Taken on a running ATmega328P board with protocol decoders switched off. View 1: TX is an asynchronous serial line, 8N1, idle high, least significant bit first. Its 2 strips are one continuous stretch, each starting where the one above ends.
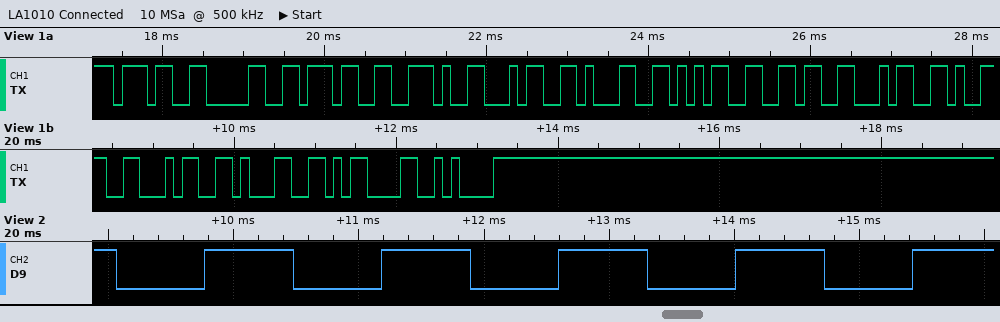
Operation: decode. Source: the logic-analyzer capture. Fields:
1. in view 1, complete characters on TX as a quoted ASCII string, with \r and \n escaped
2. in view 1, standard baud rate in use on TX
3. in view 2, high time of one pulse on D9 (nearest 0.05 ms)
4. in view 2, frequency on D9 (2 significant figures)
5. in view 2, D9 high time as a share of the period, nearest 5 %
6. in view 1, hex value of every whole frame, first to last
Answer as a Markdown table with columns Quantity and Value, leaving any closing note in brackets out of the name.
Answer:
| Quantity | Value |
|---|---|
| in view 1, complete characters on TX as a quoted ASCII string, with \r and \n escaped | "707.41564941\r\n" |
| in view 1, standard baud rate in use on TX | 9600 baud |
| in view 2, high time of one pulse on D9 | 0.70 ms |
| in view 2, frequency on D9 | 710 Hz |
| in view 2, D9 high time as a share of the period, nearest 5 % | 50 % |
| in view 1, hex value of every whole frame, first to last | 0x37 0x30 0x37 0x2E 0x34 0x31 0x35 0x36 0x34 0x39 0x34 0x31 0x0D 0x0A |
